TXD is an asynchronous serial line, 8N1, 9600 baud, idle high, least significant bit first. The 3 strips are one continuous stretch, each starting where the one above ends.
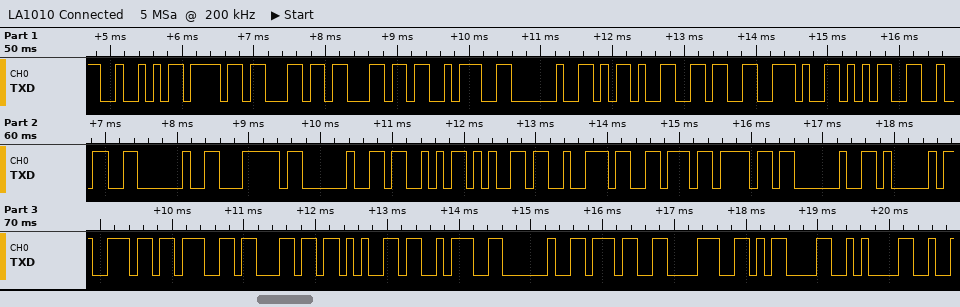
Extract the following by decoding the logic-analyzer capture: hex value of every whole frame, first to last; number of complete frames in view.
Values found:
52 6F 6C 6C 3A 20 2D 36 2E 35 32 20 7C 20 53 65 72 76 6F 20 41 6E 67 6C 65 3A 20 37 38 0D 0A
31
